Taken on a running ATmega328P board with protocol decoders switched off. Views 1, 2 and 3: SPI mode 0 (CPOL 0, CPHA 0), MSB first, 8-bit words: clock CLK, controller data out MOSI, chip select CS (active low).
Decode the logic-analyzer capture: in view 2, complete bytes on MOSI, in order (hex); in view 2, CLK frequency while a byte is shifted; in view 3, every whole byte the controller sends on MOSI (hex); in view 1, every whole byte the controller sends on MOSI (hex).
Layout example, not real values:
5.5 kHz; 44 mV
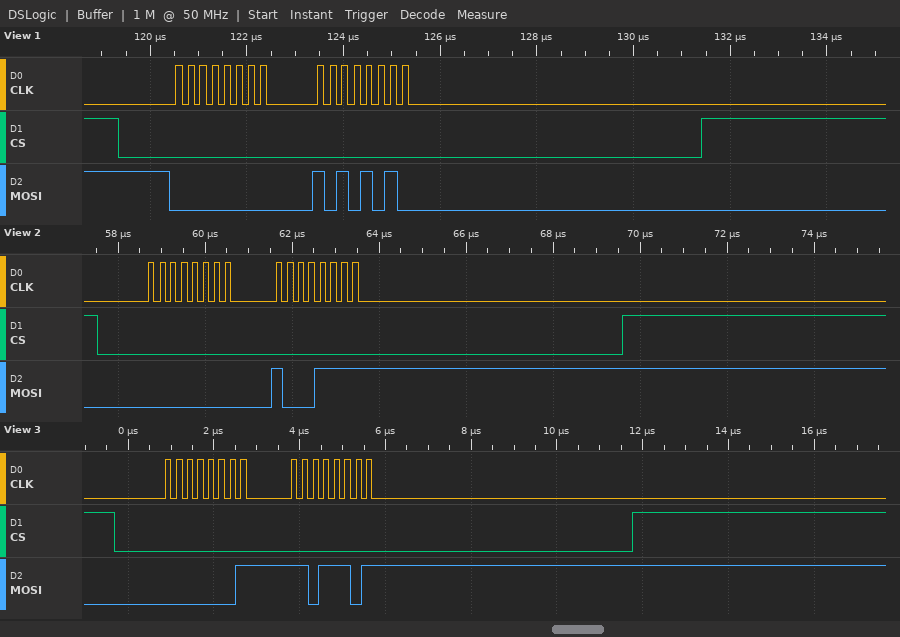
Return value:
0x00 0x8F; 4 MHz; 01 DD; 0x00 0xAA
